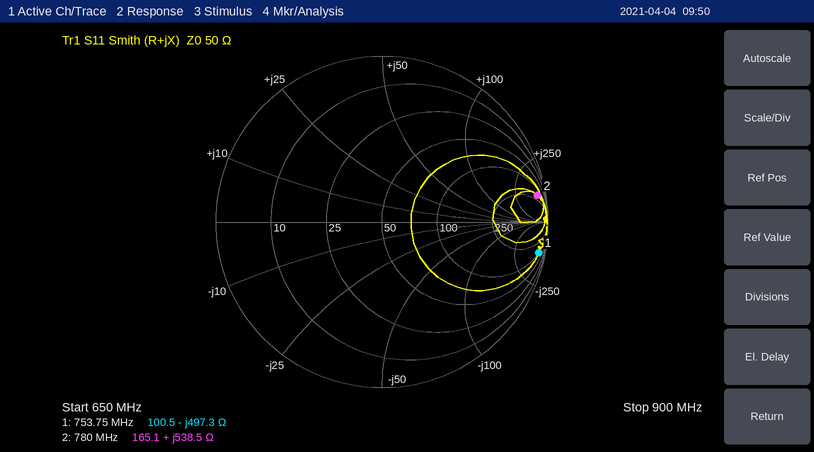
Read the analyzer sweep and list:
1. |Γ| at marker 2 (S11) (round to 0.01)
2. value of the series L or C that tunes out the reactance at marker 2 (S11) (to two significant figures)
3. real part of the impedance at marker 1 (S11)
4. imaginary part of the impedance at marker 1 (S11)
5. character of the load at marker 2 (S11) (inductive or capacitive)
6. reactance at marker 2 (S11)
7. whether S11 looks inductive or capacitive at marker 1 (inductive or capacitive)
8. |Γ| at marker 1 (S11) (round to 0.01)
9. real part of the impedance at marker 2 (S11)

0.95
380 fF
100.5 Ω
-497.3 Ω
inductive
+538.5 Ω
capacitive
0.96
165.1 Ω
